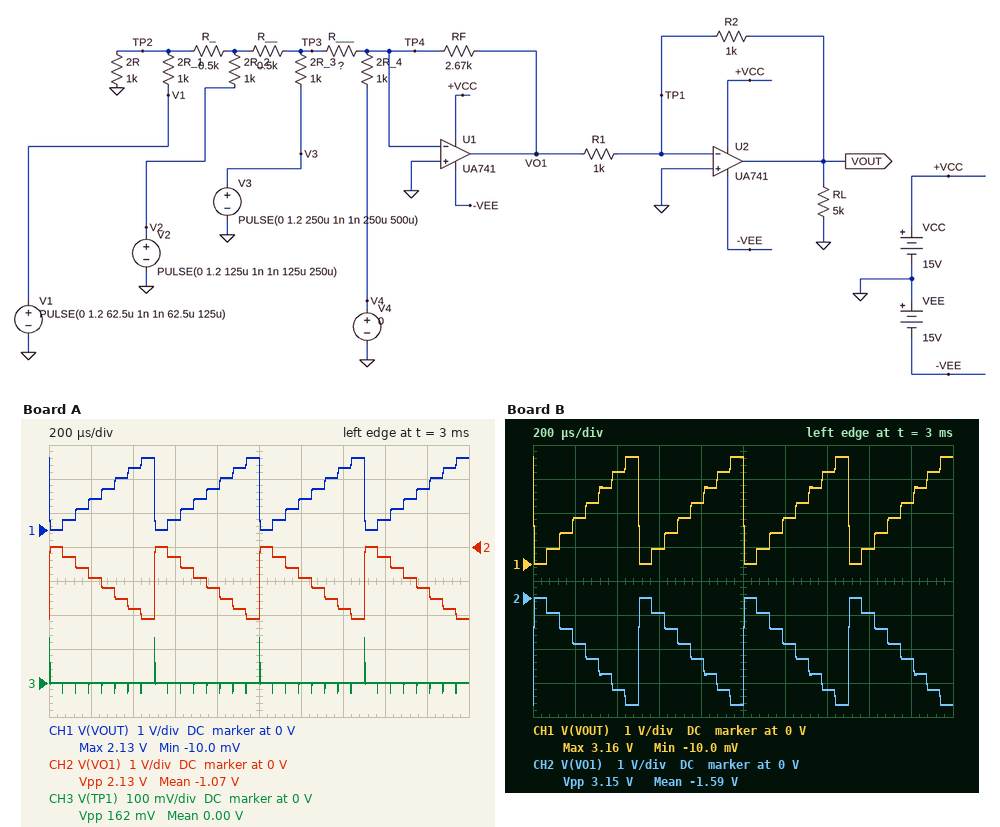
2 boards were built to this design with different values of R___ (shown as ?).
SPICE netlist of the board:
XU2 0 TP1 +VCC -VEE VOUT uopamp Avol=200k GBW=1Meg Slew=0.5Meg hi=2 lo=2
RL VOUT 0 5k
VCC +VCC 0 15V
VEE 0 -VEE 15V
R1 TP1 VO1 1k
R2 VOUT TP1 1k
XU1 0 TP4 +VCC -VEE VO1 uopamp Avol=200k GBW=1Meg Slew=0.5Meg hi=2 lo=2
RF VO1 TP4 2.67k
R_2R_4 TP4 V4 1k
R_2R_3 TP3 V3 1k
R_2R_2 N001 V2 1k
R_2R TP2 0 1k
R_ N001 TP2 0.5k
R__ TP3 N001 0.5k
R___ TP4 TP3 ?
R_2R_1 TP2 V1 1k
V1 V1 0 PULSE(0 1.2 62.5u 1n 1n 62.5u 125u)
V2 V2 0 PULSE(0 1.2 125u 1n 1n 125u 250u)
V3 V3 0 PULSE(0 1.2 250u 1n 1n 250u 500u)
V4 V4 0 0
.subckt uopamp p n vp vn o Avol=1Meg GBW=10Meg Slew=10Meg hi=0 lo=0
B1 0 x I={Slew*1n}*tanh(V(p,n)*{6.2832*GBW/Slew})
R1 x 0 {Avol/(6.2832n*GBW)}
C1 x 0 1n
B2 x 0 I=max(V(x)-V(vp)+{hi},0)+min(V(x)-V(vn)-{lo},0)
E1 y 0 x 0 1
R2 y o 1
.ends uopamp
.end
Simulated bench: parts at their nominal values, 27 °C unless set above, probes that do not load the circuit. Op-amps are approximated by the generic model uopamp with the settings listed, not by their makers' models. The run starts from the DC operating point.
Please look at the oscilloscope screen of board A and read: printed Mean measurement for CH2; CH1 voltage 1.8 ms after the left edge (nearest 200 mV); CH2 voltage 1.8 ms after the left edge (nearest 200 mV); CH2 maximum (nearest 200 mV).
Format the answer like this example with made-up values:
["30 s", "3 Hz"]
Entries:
["-1.07 V", "1.2 V", "-1.2 V", "0 V"]
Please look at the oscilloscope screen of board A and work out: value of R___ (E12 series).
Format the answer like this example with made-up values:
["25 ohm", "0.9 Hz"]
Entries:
["820 Ω"]
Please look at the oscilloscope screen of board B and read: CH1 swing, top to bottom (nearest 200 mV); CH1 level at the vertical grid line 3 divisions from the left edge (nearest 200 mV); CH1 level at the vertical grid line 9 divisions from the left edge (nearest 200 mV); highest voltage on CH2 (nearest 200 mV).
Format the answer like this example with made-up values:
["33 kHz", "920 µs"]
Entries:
["3.2 V", "400 mV", "1.8 V", "0 V"]
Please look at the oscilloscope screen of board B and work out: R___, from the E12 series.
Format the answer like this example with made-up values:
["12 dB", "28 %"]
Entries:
["390 Ω"]
